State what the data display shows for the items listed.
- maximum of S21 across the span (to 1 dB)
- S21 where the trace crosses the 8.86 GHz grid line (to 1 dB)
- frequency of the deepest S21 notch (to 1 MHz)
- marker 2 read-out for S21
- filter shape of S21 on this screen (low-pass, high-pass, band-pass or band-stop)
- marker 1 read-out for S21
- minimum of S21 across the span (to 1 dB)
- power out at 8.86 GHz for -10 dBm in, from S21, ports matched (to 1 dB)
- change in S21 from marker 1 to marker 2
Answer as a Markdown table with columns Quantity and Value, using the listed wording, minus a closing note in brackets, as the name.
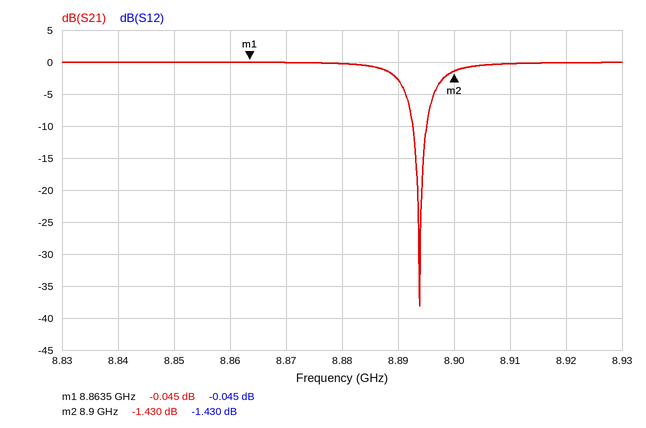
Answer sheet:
| Quantity | Value |
|---|---|
| maximum of S21 across the span | 0 dB |
| S21 where the trace crosses the 8.86 GHz grid line | 0 dB |
| frequency of the deepest S21 notch | 8.894 GHz |
| marker 2 read-out for S21 | -1.430 dB |
| filter shape of S21 on this screen | band-stop |
| marker 1 read-out for S21 | -0.045 dB |
| minimum of S21 across the span | -38 dB |
| power out at 8.86 GHz for -10 dBm in, from S21, ports matched | -10 dBm |
| change in S21 from marker 1 to marker 2 | -1.385 dB |
